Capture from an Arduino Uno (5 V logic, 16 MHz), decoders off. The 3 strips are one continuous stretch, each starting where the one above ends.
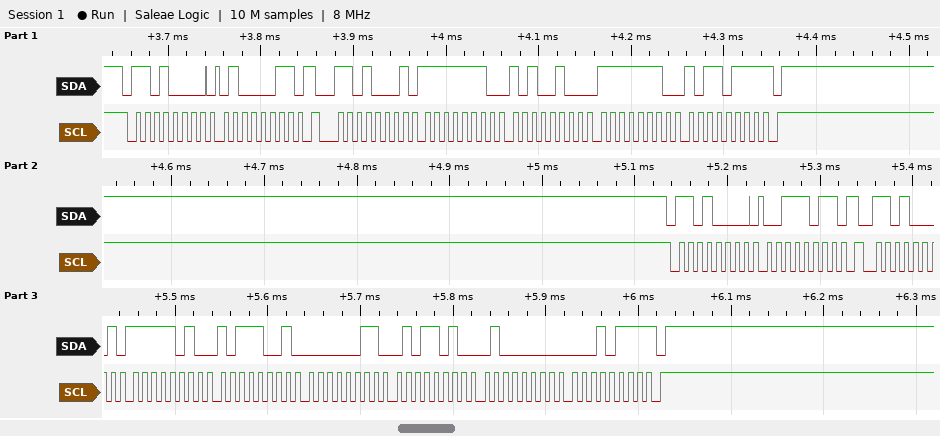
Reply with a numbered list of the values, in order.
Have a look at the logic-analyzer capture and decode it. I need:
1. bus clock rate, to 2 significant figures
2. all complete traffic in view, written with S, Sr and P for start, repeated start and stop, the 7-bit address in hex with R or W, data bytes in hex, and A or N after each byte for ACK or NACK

1. 100 kHz
2. S 68W A 43 A Sr 68R A FE A A4 A FE A B7 N P S 68W A 3B A Sr 68R A FA A B9 A 03 A 5A A 40 A 17 N P
